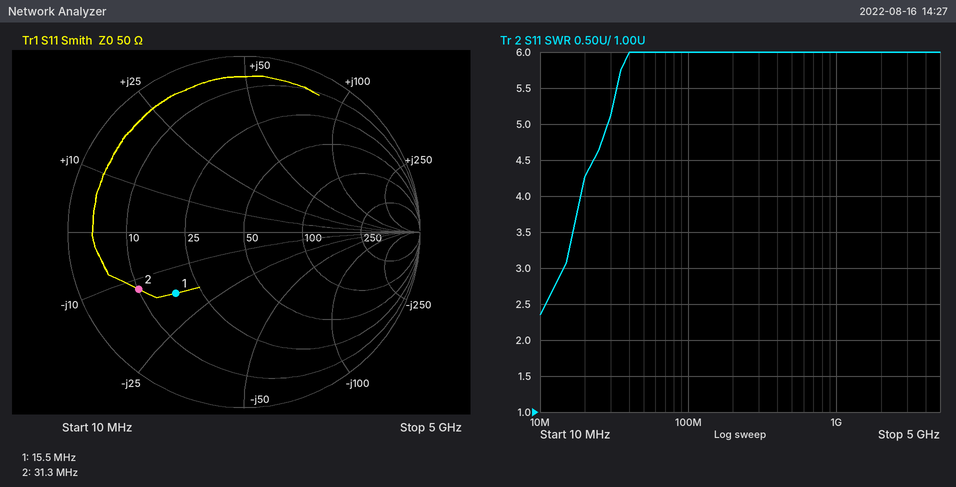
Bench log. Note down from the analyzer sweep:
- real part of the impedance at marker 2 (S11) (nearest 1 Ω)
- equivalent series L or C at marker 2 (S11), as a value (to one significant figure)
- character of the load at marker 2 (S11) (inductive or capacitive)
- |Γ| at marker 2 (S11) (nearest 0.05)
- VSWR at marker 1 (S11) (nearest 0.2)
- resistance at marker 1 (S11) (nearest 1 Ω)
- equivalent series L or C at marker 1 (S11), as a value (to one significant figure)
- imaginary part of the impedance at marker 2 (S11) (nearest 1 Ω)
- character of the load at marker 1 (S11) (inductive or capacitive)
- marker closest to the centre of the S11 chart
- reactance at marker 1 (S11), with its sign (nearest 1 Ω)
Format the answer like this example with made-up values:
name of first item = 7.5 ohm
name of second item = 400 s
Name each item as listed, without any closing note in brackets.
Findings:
real part of the impedance at marker 2 (S11) = 10 Ω
equivalent series L or C at marker 2 (S11), as a value = 400 pF
character of the load at marker 2 (S11) = capacitive
|Γ| at marker 2 (S11) = 0.70
VSWR at marker 1 (S11) = 3.2
resistance at marker 1 (S11) = 18 Ω
equivalent series L or C at marker 1 (S11), as a value = 600 pF
imaginary part of the impedance at marker 2 (S11) = -12 Ω
character of the load at marker 1 (S11) = capacitive
marker closest to the centre of the S11 chart = marker 1
reactance at marker 1 (S11), with its sign = -17 Ω
